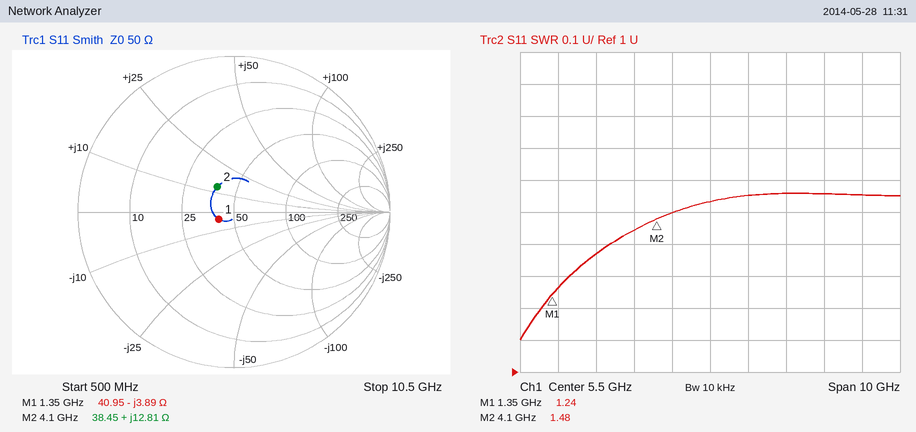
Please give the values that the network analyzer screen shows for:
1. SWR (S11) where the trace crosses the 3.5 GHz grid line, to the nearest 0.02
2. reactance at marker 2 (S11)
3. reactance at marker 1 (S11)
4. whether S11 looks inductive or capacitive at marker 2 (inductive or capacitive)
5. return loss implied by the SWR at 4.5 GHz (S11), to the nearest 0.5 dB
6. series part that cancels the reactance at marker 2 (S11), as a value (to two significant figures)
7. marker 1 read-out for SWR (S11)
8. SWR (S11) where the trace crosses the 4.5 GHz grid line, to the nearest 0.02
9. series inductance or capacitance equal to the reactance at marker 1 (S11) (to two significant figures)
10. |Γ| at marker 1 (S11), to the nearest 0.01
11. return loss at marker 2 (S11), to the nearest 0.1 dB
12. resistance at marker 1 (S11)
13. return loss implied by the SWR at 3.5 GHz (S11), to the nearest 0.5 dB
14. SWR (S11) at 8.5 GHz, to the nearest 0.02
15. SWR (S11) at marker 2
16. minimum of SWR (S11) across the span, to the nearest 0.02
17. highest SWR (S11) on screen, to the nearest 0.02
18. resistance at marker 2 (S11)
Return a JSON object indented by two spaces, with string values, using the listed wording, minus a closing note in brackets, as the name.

{
  "SWR (S11) where the trace crosses the 3.5 GHz grid line, to the nearest 0.02": "1.44",
  "reactance at marker 2": "+12.81 Ω",
  "reactance at marker 1": "-3.89 Ω",
  "whether S11 looks inductive or capacitive at marker 2": "inductive",
  "return loss implied by the SWR at 4.5 GHz (S11), to the nearest 0.5 dB": "14.0 dB",
  "series part that cancels the reactance at marker 2 (S11), as a value": "3.0 pF",
  "marker 1 read-out for SWR": "1.24",
  "SWR (S11) where the trace crosses the 4.5 GHz grid line, to the nearest 0.02": "1.50",
  "series inductance or capacitance equal to the reactance at marker 1 (S11)": "30 pF",
  "|Γ| at marker 1 (S11), to the nearest 0.01": "0.11",
  "return loss at marker 2 (S11), to the nearest 0.1 dB": "14.3 dB",
  "resistance at marker 1": "40.95 Ω",
  "return loss implied by the SWR at 3.5 GHz (S11), to the nearest 0.5 dB": "15.0 dB",
  "SWR (S11) at 8.5 GHz, to the nearest 0.02": "1.56",
  "SWR (S11) at marker 2": "1.48",
  "minimum of SWR (S11) across the span, to the nearest 0.02": "1.10",
  "highest SWR (S11) on screen, to the nearest 0.02": "1.56",
  "resistance at marker 2": "38.45 Ω"
}
